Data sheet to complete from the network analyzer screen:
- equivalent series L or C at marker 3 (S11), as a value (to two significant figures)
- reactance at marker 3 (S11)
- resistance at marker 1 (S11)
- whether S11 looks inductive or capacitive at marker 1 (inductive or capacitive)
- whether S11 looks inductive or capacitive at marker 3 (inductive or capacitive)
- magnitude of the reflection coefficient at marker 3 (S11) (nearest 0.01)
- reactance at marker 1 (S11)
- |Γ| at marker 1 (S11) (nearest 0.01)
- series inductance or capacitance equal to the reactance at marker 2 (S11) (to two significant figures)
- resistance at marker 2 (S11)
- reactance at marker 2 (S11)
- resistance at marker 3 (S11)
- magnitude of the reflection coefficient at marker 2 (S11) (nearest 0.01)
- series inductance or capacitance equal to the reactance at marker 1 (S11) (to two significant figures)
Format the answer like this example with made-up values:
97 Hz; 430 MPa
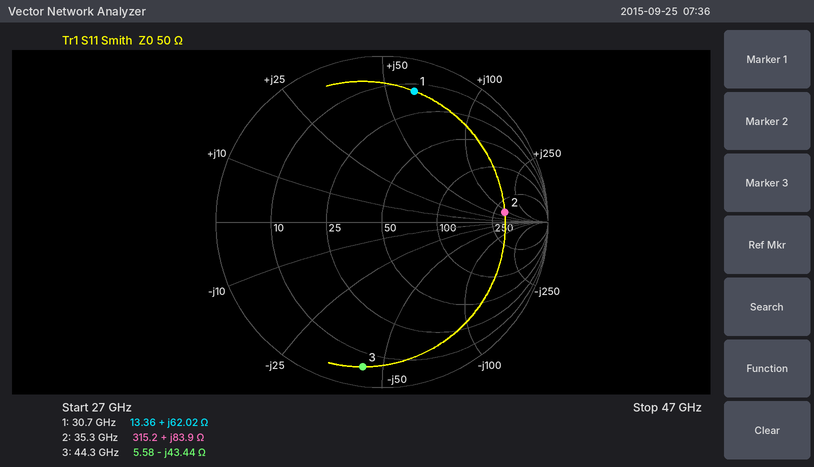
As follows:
83 fF; -43.44 Ω; 13.36 Ω; inductive; capacitive; 0.88; +62.02 Ω; 0.81; 380 pH; 315.2 Ω; +83.9 Ω; 5.58 Ω; 0.74; 320 pH
